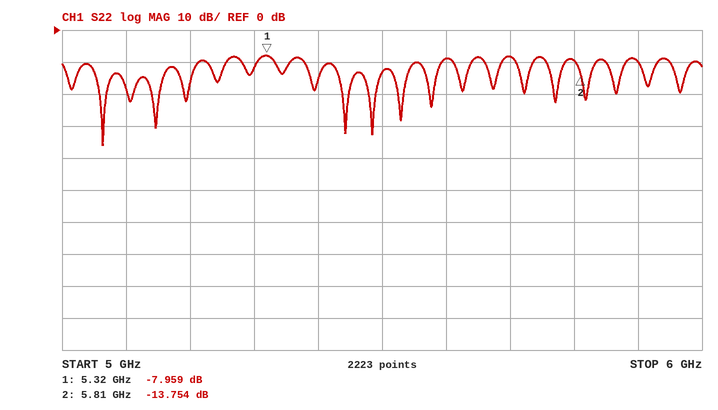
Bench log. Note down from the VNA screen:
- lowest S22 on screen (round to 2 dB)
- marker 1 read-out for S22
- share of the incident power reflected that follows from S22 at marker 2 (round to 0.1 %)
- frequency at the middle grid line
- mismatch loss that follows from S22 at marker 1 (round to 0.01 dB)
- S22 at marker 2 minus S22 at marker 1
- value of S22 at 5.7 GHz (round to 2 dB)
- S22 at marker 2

-36 dB
-7.959 dB
4.2 %
5.5 GHz
0.76 dB
-5.795 dB
-8 dB
-13.754 dB
